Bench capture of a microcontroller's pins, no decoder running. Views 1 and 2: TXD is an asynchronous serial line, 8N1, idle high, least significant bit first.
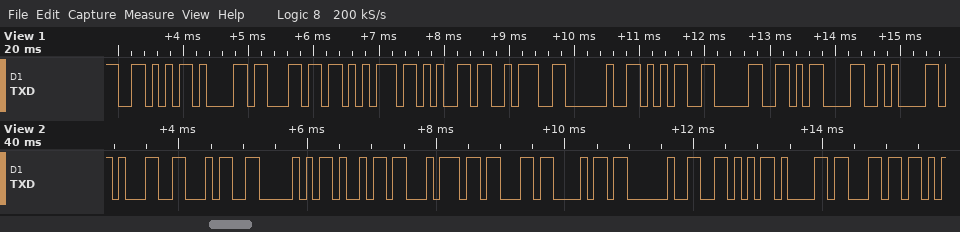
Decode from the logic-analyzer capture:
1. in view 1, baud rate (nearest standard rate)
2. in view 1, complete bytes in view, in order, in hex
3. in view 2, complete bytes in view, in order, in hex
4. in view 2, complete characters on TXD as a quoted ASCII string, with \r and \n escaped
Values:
9600 baud
56 61 6C 75 65 3A 20 35 30 0D 0A
31 34 50 69 74 63 68 20 56 61 6C
"14Pitch Val"
